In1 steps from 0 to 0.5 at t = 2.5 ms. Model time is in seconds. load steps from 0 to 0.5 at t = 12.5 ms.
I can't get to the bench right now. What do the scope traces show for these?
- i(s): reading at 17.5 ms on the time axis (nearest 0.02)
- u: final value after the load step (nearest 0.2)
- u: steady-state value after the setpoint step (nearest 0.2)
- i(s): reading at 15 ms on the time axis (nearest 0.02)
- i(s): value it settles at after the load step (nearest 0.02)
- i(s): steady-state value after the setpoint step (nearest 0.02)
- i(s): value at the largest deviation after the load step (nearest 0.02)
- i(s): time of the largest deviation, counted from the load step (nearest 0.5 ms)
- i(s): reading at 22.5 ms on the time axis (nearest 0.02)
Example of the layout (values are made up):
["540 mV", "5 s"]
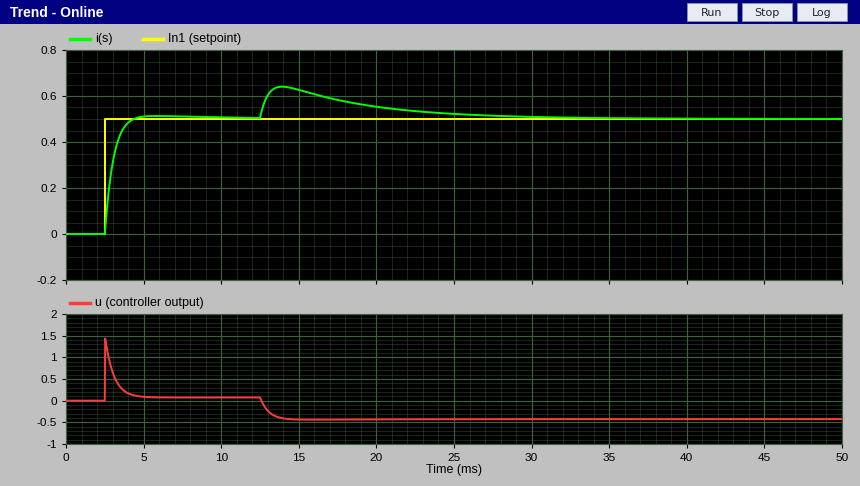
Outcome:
["0.58", "-0.4", "0.0", "0.62", "0.50", "0.50", "0.64", "1.5 ms", "0.54"]
